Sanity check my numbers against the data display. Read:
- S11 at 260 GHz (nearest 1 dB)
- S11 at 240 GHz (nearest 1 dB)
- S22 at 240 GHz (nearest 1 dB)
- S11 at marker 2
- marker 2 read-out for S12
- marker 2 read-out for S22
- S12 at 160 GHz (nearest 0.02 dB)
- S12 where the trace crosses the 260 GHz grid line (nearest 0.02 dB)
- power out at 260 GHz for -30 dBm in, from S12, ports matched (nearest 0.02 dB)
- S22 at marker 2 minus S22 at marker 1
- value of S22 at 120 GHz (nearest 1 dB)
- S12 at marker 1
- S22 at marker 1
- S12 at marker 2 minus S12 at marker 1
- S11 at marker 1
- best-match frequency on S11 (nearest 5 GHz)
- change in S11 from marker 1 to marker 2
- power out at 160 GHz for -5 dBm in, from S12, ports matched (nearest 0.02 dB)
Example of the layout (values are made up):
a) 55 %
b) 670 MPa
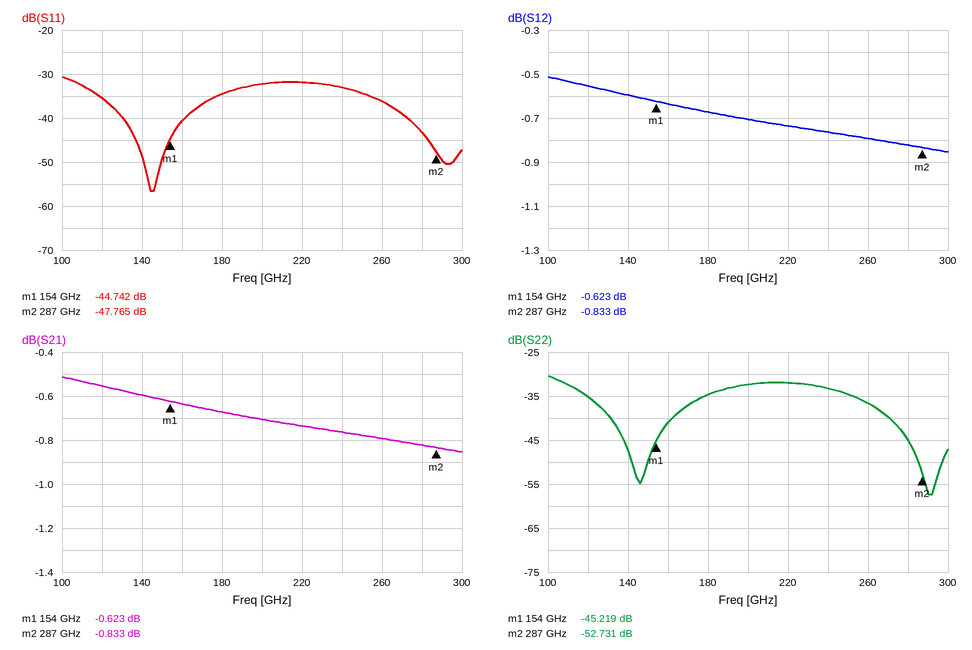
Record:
a) -36 dB
b) -33 dB
c) -33 dB
d) -47.765 dB
e) -0.833 dB
f) -52.731 dB
g) -0.64 dB
h) -0.80 dB
i) -30.80 dBm
j) -7.512 dB
k) -35 dB
l) -0.623 dB
m) -45.219 dB
n) -0.210 dB
o) -44.742 dB
p) 145 GHz
q) -3.023 dB
r) -5.64 dBm
